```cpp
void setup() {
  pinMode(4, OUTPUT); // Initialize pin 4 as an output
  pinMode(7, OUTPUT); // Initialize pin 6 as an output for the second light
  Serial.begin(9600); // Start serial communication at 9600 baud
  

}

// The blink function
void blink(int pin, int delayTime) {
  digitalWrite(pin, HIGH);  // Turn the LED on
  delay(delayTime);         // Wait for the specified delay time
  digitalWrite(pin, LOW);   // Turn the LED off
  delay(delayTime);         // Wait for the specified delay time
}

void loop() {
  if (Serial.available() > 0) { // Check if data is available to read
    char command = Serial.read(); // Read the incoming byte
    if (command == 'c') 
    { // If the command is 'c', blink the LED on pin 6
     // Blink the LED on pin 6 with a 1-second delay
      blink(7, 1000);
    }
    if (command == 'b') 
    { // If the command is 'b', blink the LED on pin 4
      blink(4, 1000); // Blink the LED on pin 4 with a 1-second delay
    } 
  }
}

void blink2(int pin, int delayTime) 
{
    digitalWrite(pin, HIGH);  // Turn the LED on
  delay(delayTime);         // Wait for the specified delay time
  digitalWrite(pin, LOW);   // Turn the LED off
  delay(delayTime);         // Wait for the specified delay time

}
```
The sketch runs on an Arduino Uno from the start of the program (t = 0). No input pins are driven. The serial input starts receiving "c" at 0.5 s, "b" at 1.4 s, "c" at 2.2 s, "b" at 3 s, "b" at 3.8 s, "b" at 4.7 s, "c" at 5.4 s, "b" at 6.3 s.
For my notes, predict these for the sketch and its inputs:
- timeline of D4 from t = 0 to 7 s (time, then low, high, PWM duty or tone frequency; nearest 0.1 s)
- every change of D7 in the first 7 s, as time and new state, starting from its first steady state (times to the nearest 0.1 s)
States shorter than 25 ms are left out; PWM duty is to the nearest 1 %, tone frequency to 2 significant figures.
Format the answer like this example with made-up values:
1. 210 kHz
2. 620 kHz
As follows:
1. 0 s low; 2.5 s high; 3.5 s low; 6.5 s high
2. 0 s low; 0.5 s high; 1.5 s low; 4.5 s high; 5.5 s low
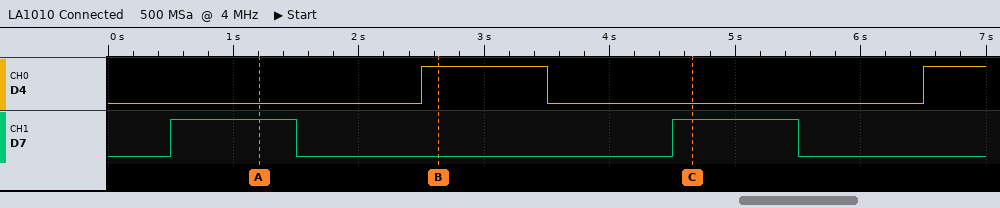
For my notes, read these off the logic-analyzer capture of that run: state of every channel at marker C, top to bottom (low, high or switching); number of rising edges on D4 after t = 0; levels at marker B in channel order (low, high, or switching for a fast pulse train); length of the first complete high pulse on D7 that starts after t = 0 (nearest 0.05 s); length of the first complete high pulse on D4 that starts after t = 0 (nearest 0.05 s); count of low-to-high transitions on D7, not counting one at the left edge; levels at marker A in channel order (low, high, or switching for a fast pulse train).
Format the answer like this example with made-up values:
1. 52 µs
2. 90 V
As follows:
1. D4 low, D7 high
2. 2
3. D4 high, D7 low
4. 1.00 s
5. 1.00 s
6. 2
7. D4 low, D7 high
